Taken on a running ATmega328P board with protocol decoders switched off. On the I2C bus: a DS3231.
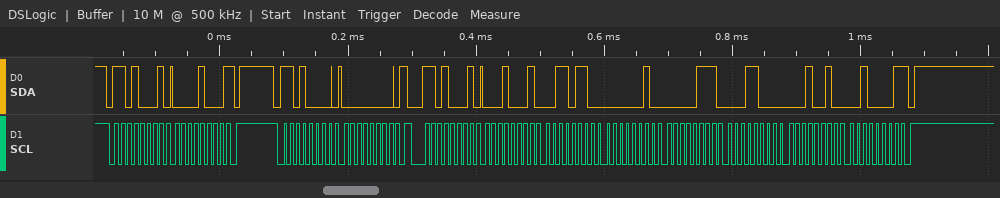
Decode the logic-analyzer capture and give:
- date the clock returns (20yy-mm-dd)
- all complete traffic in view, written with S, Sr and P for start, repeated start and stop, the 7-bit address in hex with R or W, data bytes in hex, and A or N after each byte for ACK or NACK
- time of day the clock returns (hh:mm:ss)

2021-12-18
S 68R A 08 N P S 68W A 00 A Sr 68R A 11 A 36 A 02 A 07 A 18 A 12 A 21 N P
02:36:11
